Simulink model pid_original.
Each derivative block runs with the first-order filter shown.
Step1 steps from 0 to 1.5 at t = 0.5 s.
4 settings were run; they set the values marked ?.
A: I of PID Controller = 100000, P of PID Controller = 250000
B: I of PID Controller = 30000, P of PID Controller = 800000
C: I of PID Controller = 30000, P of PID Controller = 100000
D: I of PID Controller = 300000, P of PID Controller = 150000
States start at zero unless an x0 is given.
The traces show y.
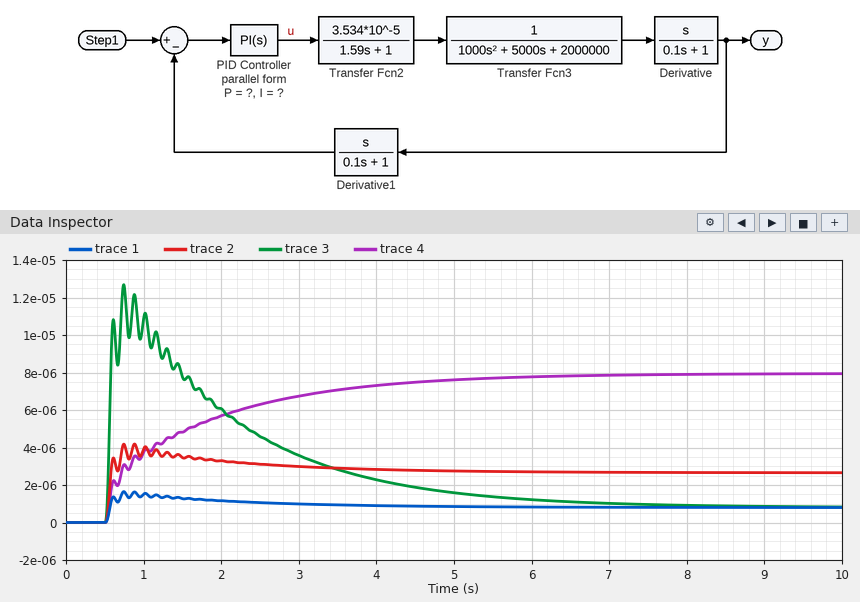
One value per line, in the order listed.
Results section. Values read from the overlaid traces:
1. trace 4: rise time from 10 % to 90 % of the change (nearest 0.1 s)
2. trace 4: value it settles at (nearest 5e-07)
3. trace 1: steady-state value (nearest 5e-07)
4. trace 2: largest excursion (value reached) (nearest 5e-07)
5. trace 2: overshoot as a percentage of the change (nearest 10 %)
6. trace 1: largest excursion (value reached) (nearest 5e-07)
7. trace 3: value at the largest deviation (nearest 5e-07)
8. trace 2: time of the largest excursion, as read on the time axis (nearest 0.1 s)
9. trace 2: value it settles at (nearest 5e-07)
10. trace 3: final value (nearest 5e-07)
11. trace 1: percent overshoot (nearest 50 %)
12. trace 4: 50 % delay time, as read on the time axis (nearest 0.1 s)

3.1 s
0.0000080
0.0000010
0.0000040
60 %
0.0000015
0.0000125
0.9 s
0.0000025
0.0000010
100 %
1.1 s
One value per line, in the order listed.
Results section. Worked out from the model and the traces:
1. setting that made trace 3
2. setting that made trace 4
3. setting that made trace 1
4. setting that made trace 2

B
D
C
A
